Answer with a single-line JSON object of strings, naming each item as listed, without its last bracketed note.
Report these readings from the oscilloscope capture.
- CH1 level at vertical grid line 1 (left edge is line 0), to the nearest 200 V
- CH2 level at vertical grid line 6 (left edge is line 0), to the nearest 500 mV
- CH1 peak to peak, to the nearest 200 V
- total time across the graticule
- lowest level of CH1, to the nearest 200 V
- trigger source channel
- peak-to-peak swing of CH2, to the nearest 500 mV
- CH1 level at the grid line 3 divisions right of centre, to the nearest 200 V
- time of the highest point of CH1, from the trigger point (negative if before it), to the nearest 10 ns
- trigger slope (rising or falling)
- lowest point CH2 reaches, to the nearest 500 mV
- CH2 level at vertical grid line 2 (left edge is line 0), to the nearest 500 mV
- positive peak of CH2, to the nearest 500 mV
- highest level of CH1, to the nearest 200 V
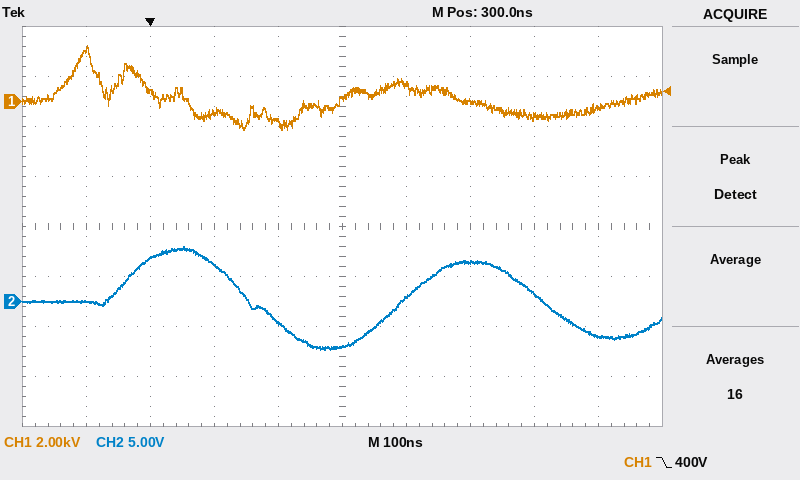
{"CH1 level at vertical grid line 1 (left edge is line 0), to the nearest 200 V": "2.0 kV", "CH2 level at vertical grid line 6 (left edge is line 0), to the nearest 500 mV": "500 mV", "CH1 peak to peak, to the nearest 200 V": "3.4 kV", "total time across the graticule": "1 µs", "lowest level of CH1, to the nearest 200 V": "-1.2 kV", "trigger source channel": "CH1", "peak-to-peak swing of CH2, to the nearest 500 mV": "10.5 V", "CH1 level at the grid line 3 divisions right of centre, to the nearest 200 V": "-600 V", "time of the highest point of CH1, from the trigger point (negative if before it), to the nearest 10 ns": "-100 ns", "trigger slope": "falling", "lowest point CH2 reaches, to the nearest 500 mV": "-5.0 V", "CH2 level at vertical grid line 2 (left edge is line 0), to the nearest 500 mV": "4.5 V", "positive peak of CH2, to the nearest 500 mV": "5.5 V", "highest level of CH1, to the nearest 200 V": "2.2 kV"}
